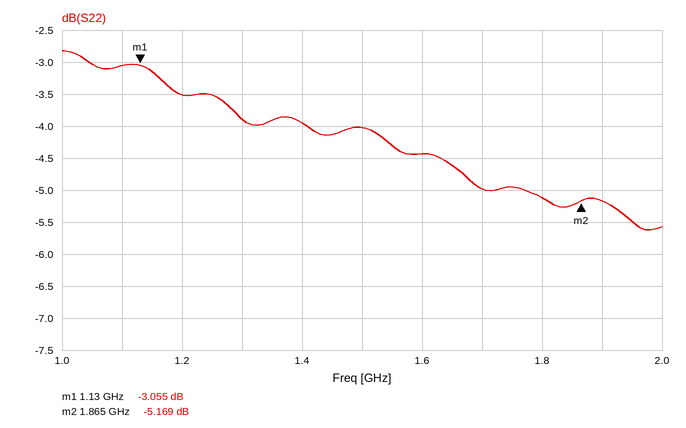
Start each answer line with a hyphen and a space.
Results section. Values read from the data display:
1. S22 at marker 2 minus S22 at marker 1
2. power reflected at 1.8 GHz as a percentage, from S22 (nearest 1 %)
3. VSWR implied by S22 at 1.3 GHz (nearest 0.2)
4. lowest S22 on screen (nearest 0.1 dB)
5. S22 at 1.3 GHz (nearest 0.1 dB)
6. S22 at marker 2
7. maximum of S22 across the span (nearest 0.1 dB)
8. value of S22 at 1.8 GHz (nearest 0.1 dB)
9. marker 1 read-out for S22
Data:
- -2.114 dB
- 31 %
- 4.6
- -5.6 dB
- -3.9 dB
- -5.169 dB
- -2.8 dB
- -5.1 dB
- -3.055 dB
